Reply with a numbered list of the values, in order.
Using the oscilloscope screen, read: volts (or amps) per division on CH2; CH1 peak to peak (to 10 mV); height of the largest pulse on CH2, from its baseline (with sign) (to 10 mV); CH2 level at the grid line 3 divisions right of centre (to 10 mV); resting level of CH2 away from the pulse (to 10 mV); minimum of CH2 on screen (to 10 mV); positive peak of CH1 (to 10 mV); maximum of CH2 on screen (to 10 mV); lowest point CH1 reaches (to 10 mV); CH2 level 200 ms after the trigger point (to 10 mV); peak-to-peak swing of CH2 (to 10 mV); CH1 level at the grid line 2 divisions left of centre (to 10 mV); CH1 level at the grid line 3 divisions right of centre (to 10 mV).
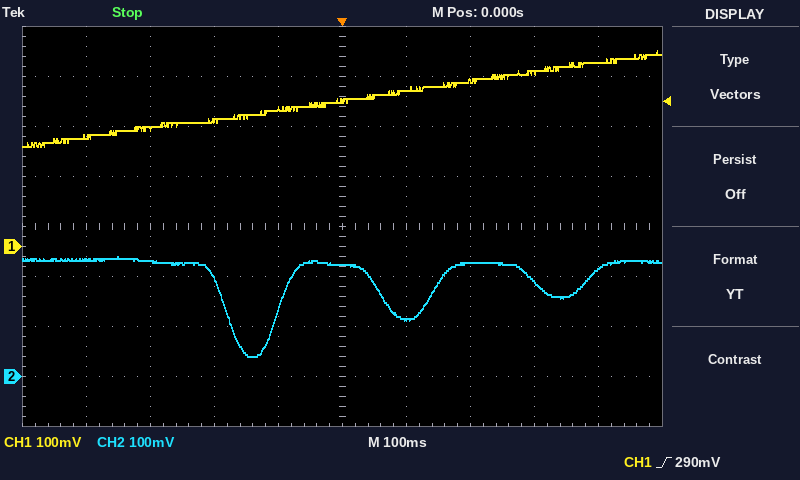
1. 100 mV
2. 190 mV
3. -190 mV
4. 190 mV
5. 230 mV
6. 40 mV
7. 390 mV
8. 240 mV
9. 200 mV
10. 230 mV
11. 200 mV
12. 250 mV
13. 350 mV
